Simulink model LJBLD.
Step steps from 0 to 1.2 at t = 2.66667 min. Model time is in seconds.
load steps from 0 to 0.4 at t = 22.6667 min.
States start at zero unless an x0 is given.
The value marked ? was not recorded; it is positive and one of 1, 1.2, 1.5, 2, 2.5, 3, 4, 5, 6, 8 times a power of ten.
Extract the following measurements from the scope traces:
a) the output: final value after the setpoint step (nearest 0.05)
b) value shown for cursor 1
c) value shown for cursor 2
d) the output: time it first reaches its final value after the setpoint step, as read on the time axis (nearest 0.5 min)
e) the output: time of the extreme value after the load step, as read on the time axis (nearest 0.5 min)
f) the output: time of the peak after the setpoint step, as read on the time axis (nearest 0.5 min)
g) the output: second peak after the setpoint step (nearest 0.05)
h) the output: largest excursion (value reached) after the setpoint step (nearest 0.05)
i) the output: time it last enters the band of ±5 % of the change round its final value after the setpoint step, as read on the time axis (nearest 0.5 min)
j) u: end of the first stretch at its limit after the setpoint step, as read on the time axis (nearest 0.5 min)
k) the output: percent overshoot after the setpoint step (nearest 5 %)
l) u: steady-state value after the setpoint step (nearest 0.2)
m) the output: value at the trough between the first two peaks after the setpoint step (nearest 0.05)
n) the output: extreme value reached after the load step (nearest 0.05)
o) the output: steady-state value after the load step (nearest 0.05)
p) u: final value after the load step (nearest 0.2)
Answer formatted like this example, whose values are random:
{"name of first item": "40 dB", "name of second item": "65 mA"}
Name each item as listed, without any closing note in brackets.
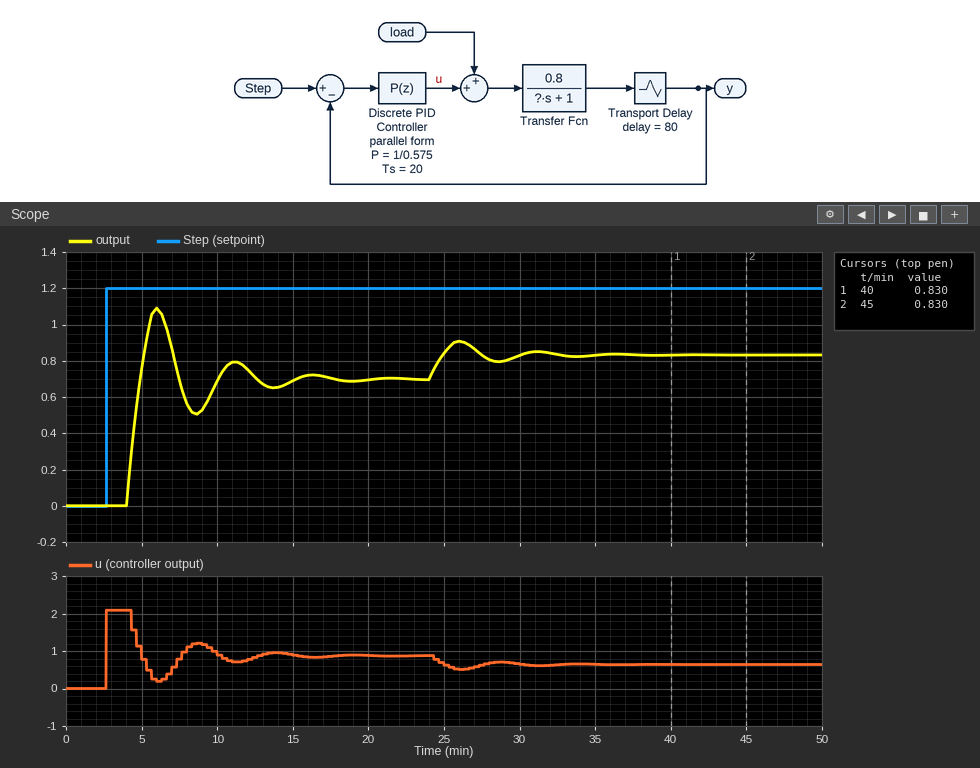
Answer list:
{"the output: final value after the setpoint step": "0.70", "value shown for cursor 1": "0.830", "value shown for cursor 2": "0.830", "the output: time it first reaches its final value after the setpoint step, as read on the time axis": "5.0 min", "the output: time of the extreme value after the load step, as read on the time axis": "26.0 min", "the output: time of the peak after the setpoint step, as read on the time axis": "6.0 min", "the output: second peak after the setpoint step": "0.80", "the output: largest excursion (value reached) after the setpoint step": "1.10", "the output: time it last enters the band of ±5 % of the change round its final value after the setpoint step, as read on the time axis": "14.5 min", "u: end of the first stretch at its limit after the setpoint step, as read on the time axis": "4.5 min", "the output: percent overshoot after the setpoint step": "55 %", "u: steady-state value after the setpoint step": "0.8", "the output: value at the trough between the first two peaks after the setpoint step": "0.50", "the output: extreme value reached after the load step": "0.90", "the output: steady-state value after the load step": "0.85", "u: final value after the load step": "0.6"}
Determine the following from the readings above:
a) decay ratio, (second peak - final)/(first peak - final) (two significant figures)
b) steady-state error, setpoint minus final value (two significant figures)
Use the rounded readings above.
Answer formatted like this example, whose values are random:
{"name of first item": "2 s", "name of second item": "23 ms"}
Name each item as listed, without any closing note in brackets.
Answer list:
{"decay ratio, (second peak - final)/(first peak - final)": "0.25", "steady-state error, setpoint minus final value": "0.50"}
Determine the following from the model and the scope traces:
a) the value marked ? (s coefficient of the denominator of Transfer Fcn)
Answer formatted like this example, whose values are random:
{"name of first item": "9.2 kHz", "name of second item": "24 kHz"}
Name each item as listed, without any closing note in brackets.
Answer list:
{"the value marked ?": "100"}
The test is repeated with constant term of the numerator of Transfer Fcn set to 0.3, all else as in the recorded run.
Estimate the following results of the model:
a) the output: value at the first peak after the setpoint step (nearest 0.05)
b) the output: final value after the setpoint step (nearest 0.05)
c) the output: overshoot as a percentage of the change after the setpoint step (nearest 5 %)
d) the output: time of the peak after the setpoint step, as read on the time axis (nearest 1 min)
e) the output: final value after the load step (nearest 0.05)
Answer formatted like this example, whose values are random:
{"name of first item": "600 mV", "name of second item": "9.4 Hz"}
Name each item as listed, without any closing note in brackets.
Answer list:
{"the output: value at the first peak after the setpoint step": "0.45", "the output: final value after the setpoint step": "0.40", "the output: overshoot as a percentage of the change after the setpoint step": "10 %", "the output: time of the peak after the setpoint step, as read on the time axis": "7 min", "the output: final value after the load step": "0.50"}
